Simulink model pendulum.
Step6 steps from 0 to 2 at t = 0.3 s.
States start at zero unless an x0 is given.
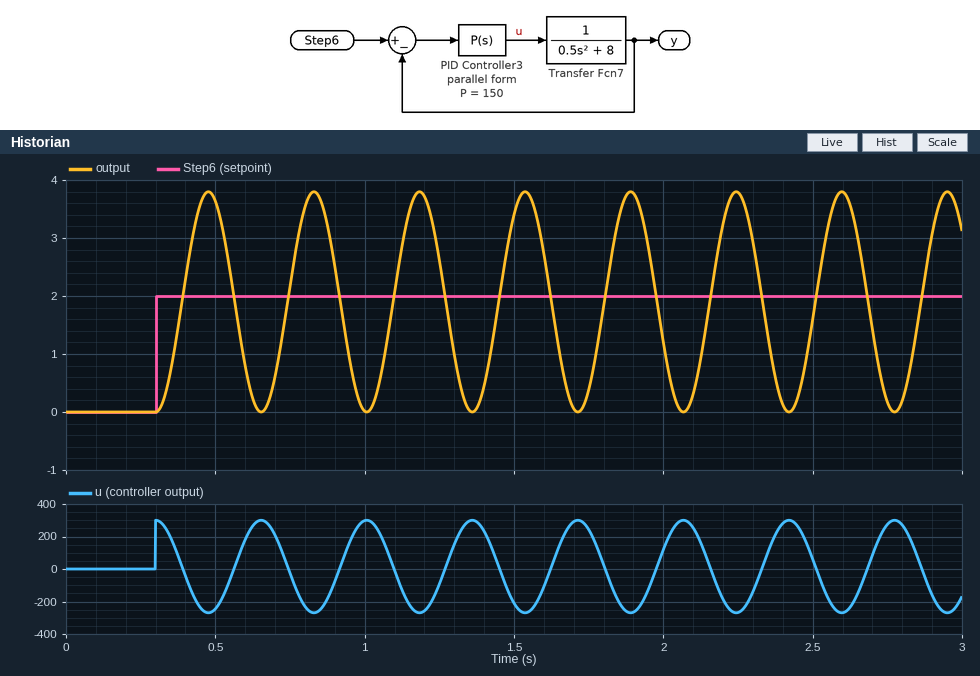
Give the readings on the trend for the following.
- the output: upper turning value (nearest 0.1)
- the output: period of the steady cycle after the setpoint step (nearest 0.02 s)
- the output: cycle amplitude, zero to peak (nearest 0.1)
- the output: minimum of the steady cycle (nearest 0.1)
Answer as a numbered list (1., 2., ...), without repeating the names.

1. 3.8
2. 0.36 s
3. 1.9
4. 0.0
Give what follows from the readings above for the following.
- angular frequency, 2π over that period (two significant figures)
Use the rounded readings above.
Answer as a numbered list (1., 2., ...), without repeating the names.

1. 17 rad/s
